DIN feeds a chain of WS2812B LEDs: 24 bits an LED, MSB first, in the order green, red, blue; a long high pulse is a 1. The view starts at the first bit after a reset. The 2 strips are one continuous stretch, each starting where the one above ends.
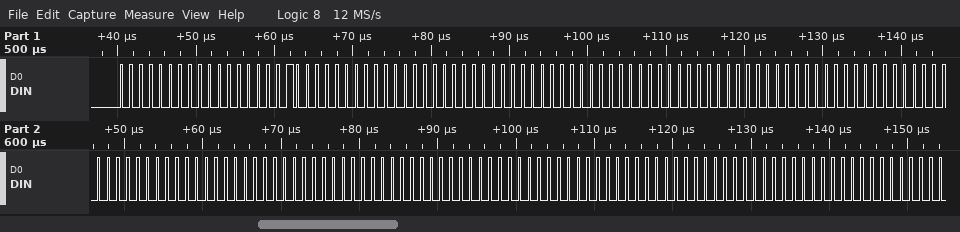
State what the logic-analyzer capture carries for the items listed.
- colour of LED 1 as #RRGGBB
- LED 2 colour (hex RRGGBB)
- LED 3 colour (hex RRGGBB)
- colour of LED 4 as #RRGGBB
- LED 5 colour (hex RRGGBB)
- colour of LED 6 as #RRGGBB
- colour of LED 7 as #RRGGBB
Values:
#000040
#000000
#000000
#000000
#000000
#000000
#000000
